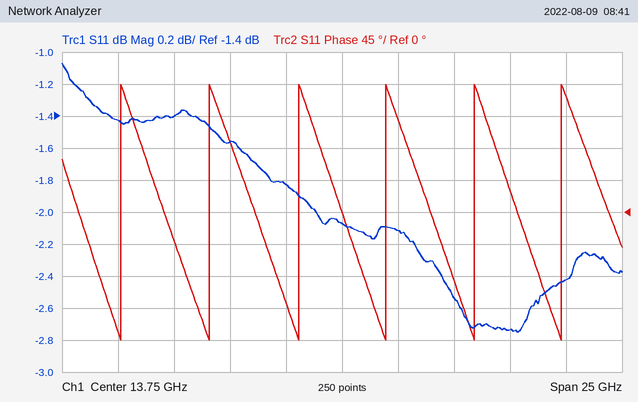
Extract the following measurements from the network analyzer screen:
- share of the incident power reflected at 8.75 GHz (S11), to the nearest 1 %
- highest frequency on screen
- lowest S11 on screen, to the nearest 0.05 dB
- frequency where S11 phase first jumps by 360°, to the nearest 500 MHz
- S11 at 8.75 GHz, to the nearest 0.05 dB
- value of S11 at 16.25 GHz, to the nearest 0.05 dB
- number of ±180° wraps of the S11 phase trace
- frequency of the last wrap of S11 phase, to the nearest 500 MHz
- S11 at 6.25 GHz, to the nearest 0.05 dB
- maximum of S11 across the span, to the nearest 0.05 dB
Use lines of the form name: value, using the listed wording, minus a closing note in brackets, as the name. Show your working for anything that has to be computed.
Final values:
share of the incident power reflected at 8.75 GHz (S11), to the nearest 1 %: 10^(-1.55/10) ≈ 70 %
highest frequency on screen: 26.25 GHz
lowest S11 on screen, to the nearest 0.05 dB: -2.75 dB
frequency where S11 phase first jumps by 360°, to the nearest 500 MHz: 4.0 GHz
S11 at 8.75 GHz, to the nearest 0.05 dB: -1.55 dB
value of S11 at 16.25 GHz, to the nearest 0.05 dB: -2.10 dB
number of ±180° wraps of the S11 phase trace: 6
frequency of the last wrap of S11 phase, to the nearest 500 MHz: 23.5 GHz
S11 at 6.25 GHz, to the nearest 0.05 dB: -1.40 dB
maximum of S11 across the span, to the nearest 0.05 dB: -1.05 dB
